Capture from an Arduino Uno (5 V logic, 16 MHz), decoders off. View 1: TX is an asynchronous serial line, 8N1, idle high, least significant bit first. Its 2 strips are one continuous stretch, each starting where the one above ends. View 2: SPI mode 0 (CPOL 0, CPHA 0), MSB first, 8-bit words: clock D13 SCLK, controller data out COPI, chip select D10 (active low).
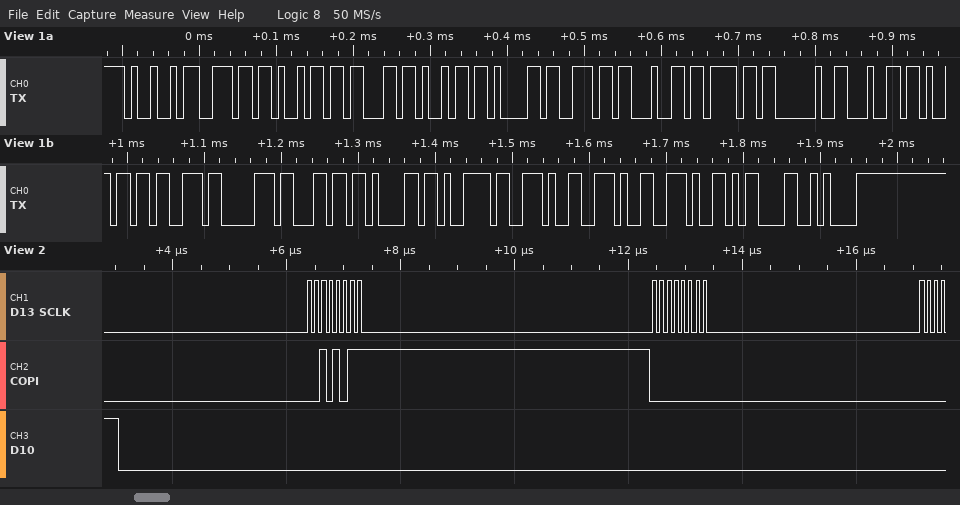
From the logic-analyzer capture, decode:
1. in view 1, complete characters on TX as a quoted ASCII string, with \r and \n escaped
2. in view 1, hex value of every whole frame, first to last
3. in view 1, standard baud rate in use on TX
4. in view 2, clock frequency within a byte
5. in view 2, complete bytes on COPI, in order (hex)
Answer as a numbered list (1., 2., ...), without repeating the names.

1. "Iniciando display...\r\n"
2. 49 6E 69 63 69 61 6E 64 6F 20 64 69 73 70 6C 61 79 2E 2E 2E 0D 0A
3. 115200 baud
4. 8 MHz
5. 2B 00
